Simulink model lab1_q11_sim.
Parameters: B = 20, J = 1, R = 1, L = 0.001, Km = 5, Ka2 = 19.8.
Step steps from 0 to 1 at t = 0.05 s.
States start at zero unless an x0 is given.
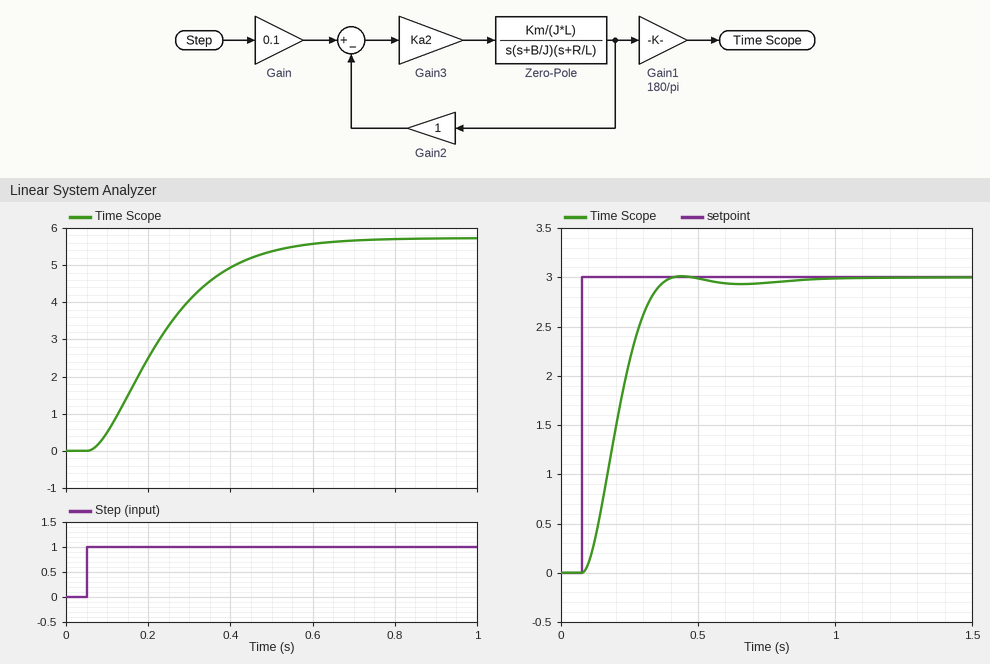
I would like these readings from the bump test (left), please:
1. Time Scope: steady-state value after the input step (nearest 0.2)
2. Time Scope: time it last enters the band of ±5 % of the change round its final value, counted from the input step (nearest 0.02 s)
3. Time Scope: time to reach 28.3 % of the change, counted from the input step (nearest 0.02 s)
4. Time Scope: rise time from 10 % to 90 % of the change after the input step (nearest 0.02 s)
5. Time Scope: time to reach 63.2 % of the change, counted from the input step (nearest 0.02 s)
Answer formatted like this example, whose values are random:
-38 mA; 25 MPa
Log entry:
5.8; 0.48 s; 0.10 s; 0.34 s; 0.22 s
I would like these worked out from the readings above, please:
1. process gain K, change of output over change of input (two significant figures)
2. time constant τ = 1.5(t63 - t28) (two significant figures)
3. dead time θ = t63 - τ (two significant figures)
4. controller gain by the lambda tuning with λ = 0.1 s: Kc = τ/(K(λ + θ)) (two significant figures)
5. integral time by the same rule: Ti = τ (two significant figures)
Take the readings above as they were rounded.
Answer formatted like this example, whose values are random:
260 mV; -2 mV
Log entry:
5.8; 0.18 s; 0.040 s; 0.22; 0.18 s
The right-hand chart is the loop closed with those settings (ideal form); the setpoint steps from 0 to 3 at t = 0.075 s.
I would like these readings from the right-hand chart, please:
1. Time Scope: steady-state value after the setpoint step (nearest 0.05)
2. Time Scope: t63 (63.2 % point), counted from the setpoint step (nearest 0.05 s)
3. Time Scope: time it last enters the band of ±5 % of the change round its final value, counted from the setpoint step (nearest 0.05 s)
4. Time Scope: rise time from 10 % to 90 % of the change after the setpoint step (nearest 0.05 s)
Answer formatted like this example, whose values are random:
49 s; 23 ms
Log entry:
3.00; 0.15 s; 0.25 s; 0.20 s
